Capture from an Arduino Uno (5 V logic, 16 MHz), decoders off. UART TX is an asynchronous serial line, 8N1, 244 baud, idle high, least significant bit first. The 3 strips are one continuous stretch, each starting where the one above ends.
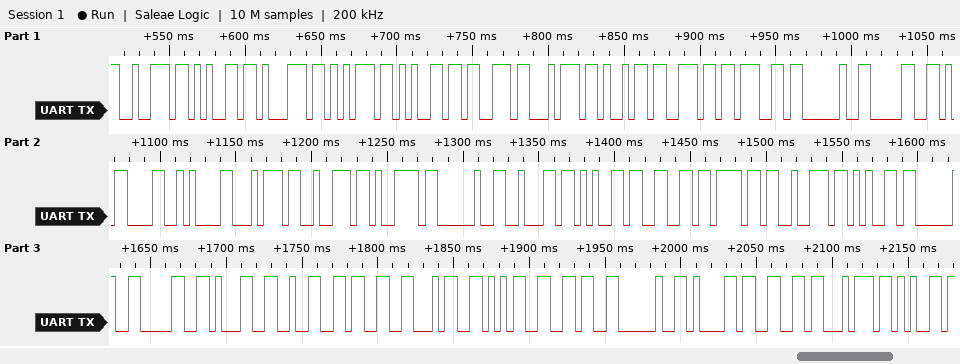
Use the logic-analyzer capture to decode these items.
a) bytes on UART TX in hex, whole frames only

72 65 71 75 65 73 74 69 6E 67 20 30 0D 0A 74 72 79 20 62 65 66 6F 72 65 20 30 31 32 33 34 35 36 20 61 66 74 65
